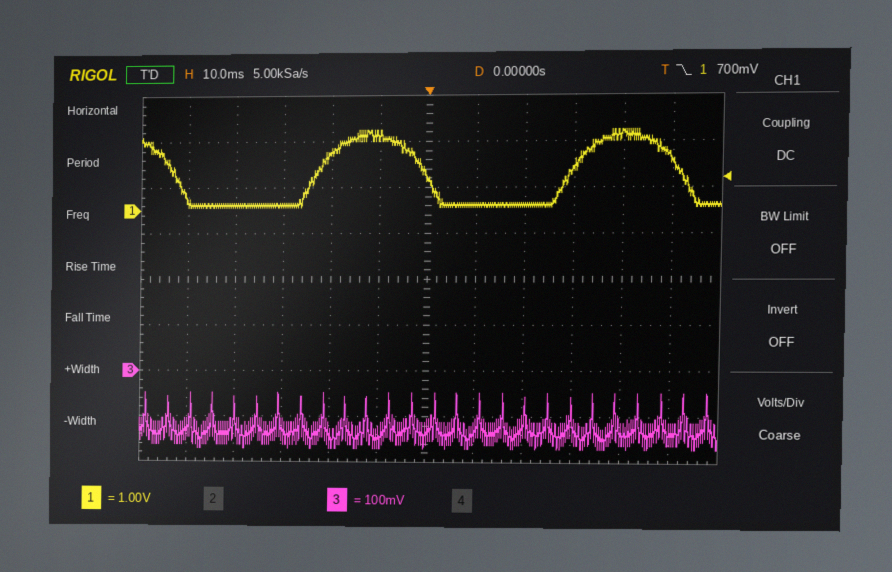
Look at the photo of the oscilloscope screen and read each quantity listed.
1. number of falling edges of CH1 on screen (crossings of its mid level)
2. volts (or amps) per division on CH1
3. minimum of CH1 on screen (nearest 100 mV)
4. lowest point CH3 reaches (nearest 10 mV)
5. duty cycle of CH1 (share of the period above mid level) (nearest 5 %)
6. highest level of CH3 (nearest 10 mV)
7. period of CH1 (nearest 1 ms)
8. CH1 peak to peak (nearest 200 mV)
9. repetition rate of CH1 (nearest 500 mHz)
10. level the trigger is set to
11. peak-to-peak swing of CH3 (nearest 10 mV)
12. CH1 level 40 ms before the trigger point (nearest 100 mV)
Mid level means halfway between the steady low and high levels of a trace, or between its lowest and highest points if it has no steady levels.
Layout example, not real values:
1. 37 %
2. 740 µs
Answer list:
1. 3
2. 1 V
3. 100 mV
4. -170 mV
5. 40 %
6. -50 mV
7. 52 ms
8. 1.6 V
9. 19.0 Hz
10. 700 mV
11. 120 mV
12. 100 mV
